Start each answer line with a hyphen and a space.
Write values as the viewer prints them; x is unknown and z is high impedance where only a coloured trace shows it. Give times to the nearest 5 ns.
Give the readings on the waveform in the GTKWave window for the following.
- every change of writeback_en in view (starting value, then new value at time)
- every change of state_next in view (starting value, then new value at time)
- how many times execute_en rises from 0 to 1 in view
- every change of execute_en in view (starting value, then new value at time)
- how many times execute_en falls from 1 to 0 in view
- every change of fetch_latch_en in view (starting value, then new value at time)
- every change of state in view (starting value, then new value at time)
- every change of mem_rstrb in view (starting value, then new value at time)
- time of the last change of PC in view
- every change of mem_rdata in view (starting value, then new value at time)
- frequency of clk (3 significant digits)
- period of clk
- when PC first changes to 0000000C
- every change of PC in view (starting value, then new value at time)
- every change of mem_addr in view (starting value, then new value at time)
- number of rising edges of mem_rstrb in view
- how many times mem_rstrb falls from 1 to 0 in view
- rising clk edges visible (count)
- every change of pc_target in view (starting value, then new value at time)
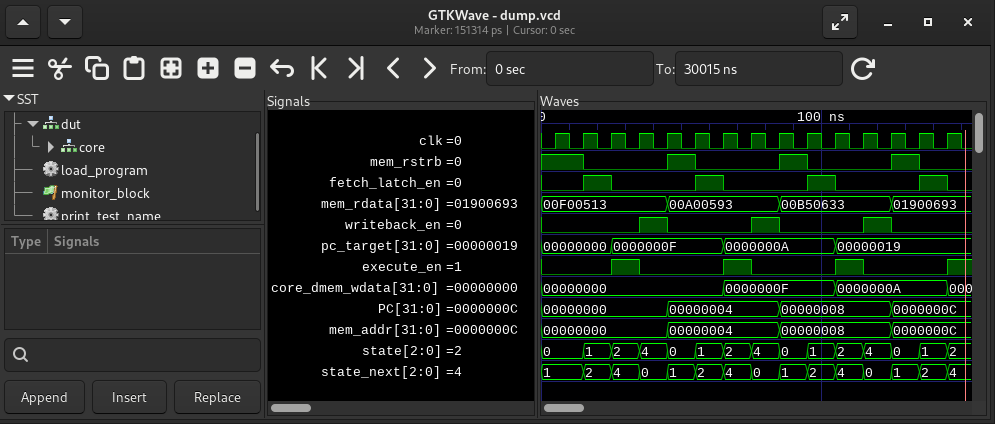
- 0, 1 at 35 ns, 0 at 45 ns, 1 at 75 ns, 0 at 85 ns, 1 at 115 ns, 0 at 125 ns
- 1, 2 at 15 ns, 4 at 25 ns, 0 at 35 ns, 1 at 45 ns, 2 at 55 ns, 4 at 65 ns, 0 at 75 ns, 1 at 85 ns, 2 at 95 ns, 4 at 105 ns, 0 at 115 ns, 1 at 125 ns, 2 at 135 ns, 4 at 145 ns
- 4
- 0, 1 at 25 ns, 0 at 35 ns, 1 at 65 ns, 0 at 75 ns, 1 at 105 ns, 0 at 115 ns, 1 at 145 ns
- 3
- 0, 1 at 15 ns, 0 at 25 ns, 1 at 55 ns, 0 at 65 ns, 1 at 95 ns, 0 at 105 ns, 1 at 135 ns, 0 at 145 ns
- 0, 1 at 15 ns, 2 at 25 ns, 4 at 35 ns, 0 at 45 ns, 1 at 55 ns, 2 at 65 ns, 4 at 75 ns, 0 at 85 ns, 1 at 95 ns, 2 at 105 ns, 4 at 115 ns, 0 at 125 ns, 1 at 135 ns, 2 at 145 ns
- 1, 0 at 15 ns, 1 at 45 ns, 0 at 55 ns, 1 at 85 ns, 0 at 95 ns, 1 at 125 ns, 0 at 135 ns
- 125 ns
- 00F00513, 00A00593 at 45 ns, 00B50633 at 85 ns, 01900693 at 125 ns
- 100 MHz
- 10 ns
- 125 ns
- 00000000, 00000004 at 45 ns, 00000008 at 85 ns, 0000000C at 125 ns
- 00000000, 00000004 at 45 ns, 00000008 at 85 ns, 0000000C at 125 ns
- 3
- 4
- 15
- 00000000, 0000000F at 25 ns, 0000000A at 65 ns, 00000019 at 105 ns
